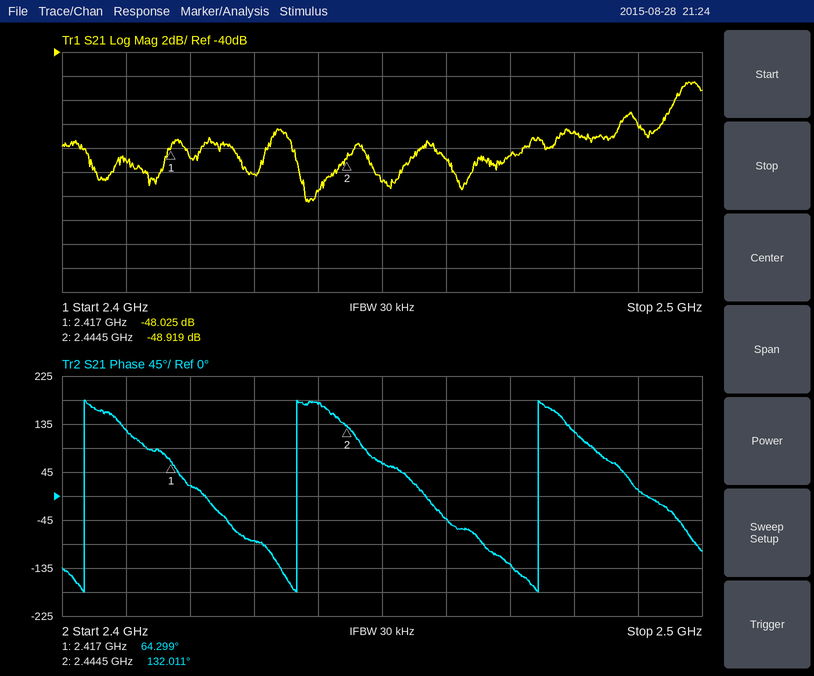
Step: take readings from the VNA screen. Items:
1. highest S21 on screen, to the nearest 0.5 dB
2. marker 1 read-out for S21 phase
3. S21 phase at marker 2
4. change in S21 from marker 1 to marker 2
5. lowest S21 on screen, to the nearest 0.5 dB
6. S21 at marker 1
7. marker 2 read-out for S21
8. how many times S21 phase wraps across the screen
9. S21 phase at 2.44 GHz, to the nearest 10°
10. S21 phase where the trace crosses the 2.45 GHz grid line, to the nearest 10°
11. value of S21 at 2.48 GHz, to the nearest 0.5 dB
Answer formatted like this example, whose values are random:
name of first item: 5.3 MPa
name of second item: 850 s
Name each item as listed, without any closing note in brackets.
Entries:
highest S21 on screen, to the nearest 0.5 dB: -42.5 dB
marker 1 read-out for S21 phase: 64.299°
S21 phase at marker 2: 132.011°
change in S21 from marker 1 to marker 2: -0.894 dB
lowest S21 on screen, to the nearest 0.5 dB: -52.5 dB
S21 at marker 1: -48.025 dB
marker 2 read-out for S21: -48.919 dB
how many times S21 phase wraps across the screen: 3
S21 phase at 2.44 GHz, to the nearest 10°: 170°
S21 phase where the trace crosses the 2.45 GHz grid line, to the nearest 10°: 60°
value of S21 at 2.48 GHz, to the nearest 0.5 dB: -46.5 dB
